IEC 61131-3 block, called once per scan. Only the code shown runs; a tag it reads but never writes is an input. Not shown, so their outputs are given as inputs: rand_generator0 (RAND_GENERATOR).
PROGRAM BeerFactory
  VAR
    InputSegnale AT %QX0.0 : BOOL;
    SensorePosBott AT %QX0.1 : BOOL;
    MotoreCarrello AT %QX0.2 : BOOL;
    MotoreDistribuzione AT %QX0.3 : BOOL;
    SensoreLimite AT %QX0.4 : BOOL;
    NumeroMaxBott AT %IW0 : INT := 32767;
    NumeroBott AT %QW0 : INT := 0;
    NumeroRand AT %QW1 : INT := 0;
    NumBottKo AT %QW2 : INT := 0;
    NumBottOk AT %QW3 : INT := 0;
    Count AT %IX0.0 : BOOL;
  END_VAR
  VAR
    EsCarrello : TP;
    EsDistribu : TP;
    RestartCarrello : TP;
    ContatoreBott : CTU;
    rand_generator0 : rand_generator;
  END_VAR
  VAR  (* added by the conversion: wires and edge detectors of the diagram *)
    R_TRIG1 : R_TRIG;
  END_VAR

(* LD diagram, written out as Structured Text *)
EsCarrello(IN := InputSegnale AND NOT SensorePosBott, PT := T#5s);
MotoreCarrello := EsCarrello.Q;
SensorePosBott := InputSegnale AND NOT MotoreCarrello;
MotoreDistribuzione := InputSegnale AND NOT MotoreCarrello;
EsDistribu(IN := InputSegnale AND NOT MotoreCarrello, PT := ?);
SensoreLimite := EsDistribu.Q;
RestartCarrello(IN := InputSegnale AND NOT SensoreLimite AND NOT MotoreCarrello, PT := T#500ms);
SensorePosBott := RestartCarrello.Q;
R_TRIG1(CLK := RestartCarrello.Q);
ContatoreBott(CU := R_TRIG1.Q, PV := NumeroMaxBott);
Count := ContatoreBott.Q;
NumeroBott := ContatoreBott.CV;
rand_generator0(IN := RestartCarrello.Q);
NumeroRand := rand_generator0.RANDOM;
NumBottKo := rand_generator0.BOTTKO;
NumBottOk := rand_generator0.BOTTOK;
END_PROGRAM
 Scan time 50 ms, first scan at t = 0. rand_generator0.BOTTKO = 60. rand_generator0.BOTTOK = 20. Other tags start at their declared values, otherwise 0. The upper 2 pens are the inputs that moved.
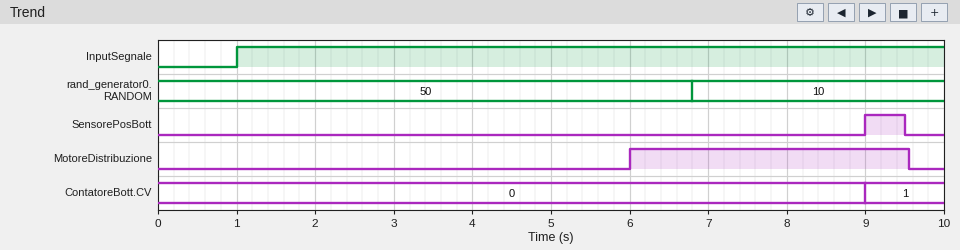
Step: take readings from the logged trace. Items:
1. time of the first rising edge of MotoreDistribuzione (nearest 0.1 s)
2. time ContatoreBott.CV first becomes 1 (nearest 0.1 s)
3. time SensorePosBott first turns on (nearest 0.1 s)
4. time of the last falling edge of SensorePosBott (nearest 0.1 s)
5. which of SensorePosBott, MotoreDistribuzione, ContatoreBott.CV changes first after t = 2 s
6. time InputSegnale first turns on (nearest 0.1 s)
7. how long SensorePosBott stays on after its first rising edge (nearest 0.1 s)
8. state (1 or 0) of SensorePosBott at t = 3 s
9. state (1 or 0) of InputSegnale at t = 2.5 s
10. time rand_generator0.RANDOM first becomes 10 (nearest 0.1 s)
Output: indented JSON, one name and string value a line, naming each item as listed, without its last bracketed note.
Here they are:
{
  "time of the first rising edge of MotoreDistribuzione": "6.0 s",
  "time ContatoreBott.CV first becomes 1": "9.0 s",
  "time SensorePosBott first turns on": "9.0 s",
  "time of the last falling edge of SensorePosBott": "9.5 s",
  "which of SensorePosBott, MotoreDistribuzione, ContatoreBott.CV changes first after t = 2 s": "MotoreDistribuzione",
  "time InputSegnale first turns on": "1.0 s",
  "how long SensorePosBott stays on after its first rising edge": "0.5 s",
  "state (1 or 0) of SensorePosBott at t = 3 s": "0",
  "state (1 or 0) of InputSegnale at t = 2.5 s": "1",
  "time rand_generator0.RANDOM first becomes 10": "6.8 s"
}
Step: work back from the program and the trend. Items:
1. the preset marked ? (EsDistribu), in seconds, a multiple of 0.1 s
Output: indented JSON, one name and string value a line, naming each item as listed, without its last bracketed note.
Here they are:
{
  "the preset marked ? (EsDistribu), in seconds, a multiple of 0.1 s": "3.0 s"
}
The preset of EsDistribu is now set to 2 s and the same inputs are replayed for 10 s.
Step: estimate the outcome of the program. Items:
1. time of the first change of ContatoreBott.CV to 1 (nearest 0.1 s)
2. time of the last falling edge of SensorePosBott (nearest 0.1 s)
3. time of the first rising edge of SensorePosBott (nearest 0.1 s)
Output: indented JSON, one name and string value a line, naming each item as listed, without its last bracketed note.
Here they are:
{
  "time of the first change of ContatoreBott.CV to 1": "8.0 s",
  "time of the last falling edge of SensorePosBott": "8.5 s",
  "time of the first rising edge of SensorePosBott": "8.0 s"
}
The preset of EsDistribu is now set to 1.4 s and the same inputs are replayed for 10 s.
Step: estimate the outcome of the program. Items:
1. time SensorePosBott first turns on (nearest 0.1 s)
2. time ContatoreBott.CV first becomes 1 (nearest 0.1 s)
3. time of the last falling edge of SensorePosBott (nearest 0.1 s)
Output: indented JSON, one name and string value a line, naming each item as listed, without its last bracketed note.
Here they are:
{
  "time SensorePosBott first turns on": "7.4 s",
  "time ContatoreBott.CV first becomes 1": "7.4 s",
  "time of the last falling edge of SensorePosBott": "7.9 s"
}
